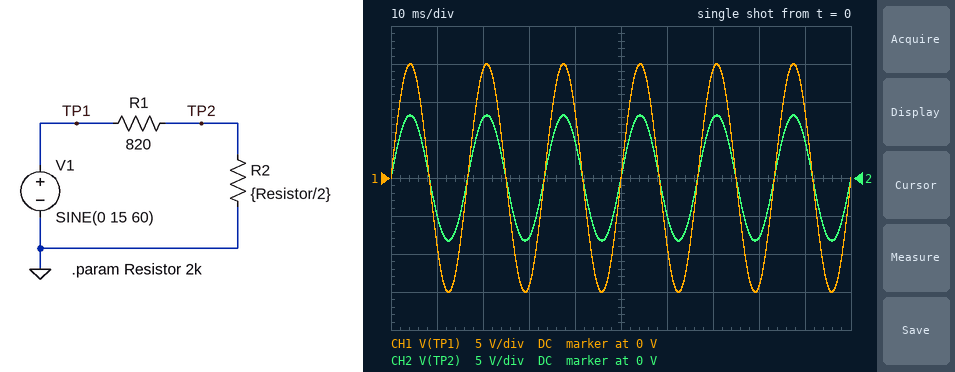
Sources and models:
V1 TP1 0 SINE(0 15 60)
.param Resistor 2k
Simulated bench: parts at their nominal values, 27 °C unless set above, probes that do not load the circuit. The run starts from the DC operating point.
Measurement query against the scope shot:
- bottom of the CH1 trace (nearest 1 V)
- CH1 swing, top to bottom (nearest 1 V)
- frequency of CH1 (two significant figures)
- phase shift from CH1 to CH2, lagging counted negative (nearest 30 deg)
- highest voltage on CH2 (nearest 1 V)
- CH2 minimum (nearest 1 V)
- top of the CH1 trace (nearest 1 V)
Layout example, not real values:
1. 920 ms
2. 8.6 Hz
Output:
1. -15 V
2. 30 V
3. 60 Hz
4. 0 deg
5. 8 V
6. -8 V
7. 15 V
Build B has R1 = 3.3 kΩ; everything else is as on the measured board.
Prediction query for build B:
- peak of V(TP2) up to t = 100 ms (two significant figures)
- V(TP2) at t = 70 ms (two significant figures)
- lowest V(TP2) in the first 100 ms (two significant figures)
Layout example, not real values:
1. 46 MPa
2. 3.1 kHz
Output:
1. 3.5 V
2. 3.3 V
3. -3.5 V
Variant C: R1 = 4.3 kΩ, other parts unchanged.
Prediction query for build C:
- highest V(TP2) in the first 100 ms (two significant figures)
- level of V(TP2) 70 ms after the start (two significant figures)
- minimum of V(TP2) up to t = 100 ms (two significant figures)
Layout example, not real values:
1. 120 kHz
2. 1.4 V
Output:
1. 2.8 V
2. 2.7 V
3. -2.8 V
